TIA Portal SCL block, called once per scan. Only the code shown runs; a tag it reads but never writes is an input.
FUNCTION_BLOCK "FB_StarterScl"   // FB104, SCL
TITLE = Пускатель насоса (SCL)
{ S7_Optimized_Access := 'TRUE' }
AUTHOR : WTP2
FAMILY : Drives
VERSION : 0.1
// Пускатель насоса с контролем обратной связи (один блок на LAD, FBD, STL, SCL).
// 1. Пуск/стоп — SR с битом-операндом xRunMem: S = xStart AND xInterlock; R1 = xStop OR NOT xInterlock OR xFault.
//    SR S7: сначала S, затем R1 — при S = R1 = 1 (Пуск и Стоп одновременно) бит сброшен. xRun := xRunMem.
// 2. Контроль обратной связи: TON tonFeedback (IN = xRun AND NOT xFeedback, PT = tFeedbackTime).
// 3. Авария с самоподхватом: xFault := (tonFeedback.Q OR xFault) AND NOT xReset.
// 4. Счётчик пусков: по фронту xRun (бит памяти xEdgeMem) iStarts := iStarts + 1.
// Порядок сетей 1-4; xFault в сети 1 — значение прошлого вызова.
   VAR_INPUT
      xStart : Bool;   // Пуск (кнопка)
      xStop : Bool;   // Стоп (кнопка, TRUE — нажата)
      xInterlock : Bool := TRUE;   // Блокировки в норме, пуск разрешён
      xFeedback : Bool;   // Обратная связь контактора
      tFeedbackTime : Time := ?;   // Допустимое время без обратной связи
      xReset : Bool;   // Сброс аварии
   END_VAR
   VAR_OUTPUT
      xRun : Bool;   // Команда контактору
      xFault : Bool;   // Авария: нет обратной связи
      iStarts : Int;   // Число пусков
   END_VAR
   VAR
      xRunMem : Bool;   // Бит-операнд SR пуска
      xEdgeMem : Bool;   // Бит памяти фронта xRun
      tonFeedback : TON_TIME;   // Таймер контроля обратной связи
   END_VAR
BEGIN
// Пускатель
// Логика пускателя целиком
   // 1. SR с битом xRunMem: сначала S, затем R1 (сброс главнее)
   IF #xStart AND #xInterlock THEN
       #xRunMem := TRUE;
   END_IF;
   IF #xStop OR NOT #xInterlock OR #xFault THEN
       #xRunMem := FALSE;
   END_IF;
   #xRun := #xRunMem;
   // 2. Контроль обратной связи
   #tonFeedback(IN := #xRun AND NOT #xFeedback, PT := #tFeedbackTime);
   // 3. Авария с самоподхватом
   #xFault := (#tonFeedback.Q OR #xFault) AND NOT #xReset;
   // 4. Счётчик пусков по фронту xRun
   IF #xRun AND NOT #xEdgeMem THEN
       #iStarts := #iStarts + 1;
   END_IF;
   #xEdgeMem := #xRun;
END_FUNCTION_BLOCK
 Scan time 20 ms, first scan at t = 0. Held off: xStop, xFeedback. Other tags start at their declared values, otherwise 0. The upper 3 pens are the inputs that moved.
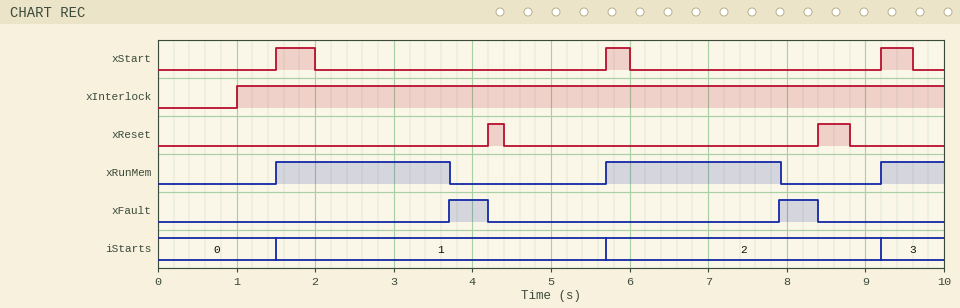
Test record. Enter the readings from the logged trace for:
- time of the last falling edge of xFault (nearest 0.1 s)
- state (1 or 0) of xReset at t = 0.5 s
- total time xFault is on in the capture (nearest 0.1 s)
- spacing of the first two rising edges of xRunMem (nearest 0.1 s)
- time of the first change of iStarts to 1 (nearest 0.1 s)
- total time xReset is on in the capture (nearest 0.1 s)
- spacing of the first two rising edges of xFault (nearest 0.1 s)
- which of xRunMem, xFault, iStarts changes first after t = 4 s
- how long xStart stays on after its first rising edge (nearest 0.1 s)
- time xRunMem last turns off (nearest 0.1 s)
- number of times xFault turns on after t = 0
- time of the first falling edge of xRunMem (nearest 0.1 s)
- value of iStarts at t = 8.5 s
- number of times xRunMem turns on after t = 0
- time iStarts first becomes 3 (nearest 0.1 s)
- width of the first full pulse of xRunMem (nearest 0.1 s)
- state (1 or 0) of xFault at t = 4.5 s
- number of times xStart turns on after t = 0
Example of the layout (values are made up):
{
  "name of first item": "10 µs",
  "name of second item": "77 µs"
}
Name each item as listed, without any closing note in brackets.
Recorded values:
{
  "time of the last falling edge of xFault": "8.4 s",
  "state (1 or 0) of xReset at t = 0.5 s": "0",
  "total time xFault is on in the capture": "1.0 s",
  "spacing of the first two rising edges of xRunMem": "4.2 s",
  "time of the first change of iStarts to 1": "1.5 s",
  "total time xReset is on in the capture": "0.6 s",
  "spacing of the first two rising edges of xFault": "4.2 s",
  "which of xRunMem, xFault, iStarts changes first after t = 4 s": "xFault",
  "how long xStart stays on after its first rising edge": "0.5 s",
  "time xRunMem last turns off": "7.9 s",
  "number of times xFault turns on after t = 0": "2",
  "time of the first falling edge of xRunMem": "3.7 s",
  "value of iStarts at t = 8.5 s": "2",
  "number of times xRunMem turns on after t = 0": "3",
  "time iStarts first becomes 3": "9.2 s",
  "width of the first full pulse of xRunMem": "2.2 s",
  "state (1 or 0) of xFault at t = 4.5 s": "0",
  "number of times xStart turns on after t = 0": "3"
}
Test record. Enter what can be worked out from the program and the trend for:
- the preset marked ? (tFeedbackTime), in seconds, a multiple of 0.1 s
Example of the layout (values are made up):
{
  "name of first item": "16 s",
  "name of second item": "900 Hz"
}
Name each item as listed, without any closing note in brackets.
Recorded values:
{
  "the preset marked ? (tFeedbackTime), in seconds, a multiple of 0.1 s": "2.2 s"
}
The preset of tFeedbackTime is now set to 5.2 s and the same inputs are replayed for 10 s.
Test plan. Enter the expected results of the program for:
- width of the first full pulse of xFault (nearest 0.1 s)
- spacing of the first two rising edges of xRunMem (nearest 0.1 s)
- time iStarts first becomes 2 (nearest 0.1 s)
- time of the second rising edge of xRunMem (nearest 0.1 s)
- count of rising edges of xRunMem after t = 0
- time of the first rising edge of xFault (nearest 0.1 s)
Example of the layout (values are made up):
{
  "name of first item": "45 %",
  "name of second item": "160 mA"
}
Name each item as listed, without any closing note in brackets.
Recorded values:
{
  "width of the first full pulse of xFault": "1.7 s",
  "spacing of the first two rising edges of xRunMem": "7.7 s",
  "time iStarts first becomes 2": "9.2 s",
  "time of the second rising edge of xRunMem": "9.2 s",
  "count of rising edges of xRunMem after t = 0": "2",
  "time of the first rising edge of xFault": "6.7 s"
}
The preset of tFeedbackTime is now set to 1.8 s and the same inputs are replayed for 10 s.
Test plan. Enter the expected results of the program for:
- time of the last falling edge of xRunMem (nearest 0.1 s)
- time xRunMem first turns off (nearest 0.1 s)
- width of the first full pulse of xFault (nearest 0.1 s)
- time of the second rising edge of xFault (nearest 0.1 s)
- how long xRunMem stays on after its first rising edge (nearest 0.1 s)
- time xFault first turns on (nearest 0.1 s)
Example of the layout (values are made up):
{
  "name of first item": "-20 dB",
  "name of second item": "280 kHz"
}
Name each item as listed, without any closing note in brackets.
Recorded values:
{
  "time of the last falling edge of xRunMem": "7.5 s",
  "time xRunMem first turns off": "3.3 s",
  "width of the first full pulse of xFault": "0.9 s",
  "time of the second rising edge of xFault": "7.5 s",
  "how long xRunMem stays on after its first rising edge": "1.8 s",
  "time xFault first turns on": "3.3 s"
}
